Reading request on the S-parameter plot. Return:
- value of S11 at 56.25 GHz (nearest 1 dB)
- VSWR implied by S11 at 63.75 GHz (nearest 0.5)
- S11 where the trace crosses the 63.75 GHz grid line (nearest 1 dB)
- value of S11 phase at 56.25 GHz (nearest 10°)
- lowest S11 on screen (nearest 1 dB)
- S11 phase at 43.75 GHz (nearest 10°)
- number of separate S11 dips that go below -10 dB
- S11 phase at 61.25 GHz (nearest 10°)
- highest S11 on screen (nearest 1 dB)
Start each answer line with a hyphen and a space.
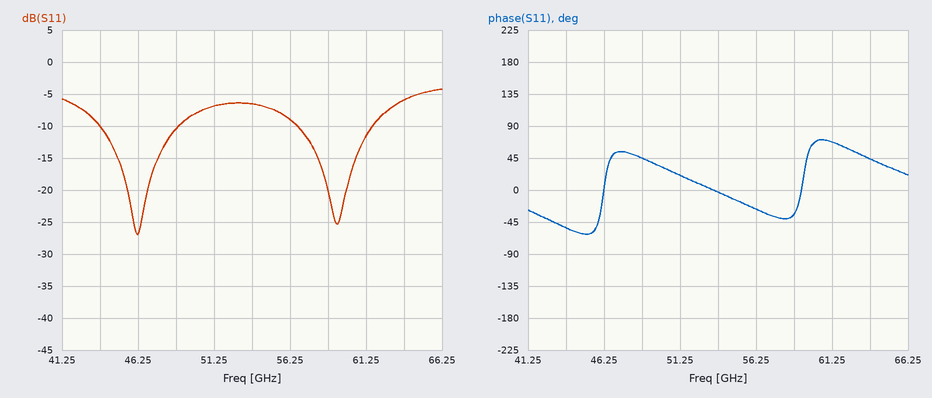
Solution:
- -9 dB
- 3.0
- -6 dB
- -30°
- -27 dB
- -50°
- 2
- 70°
- -4 dB
